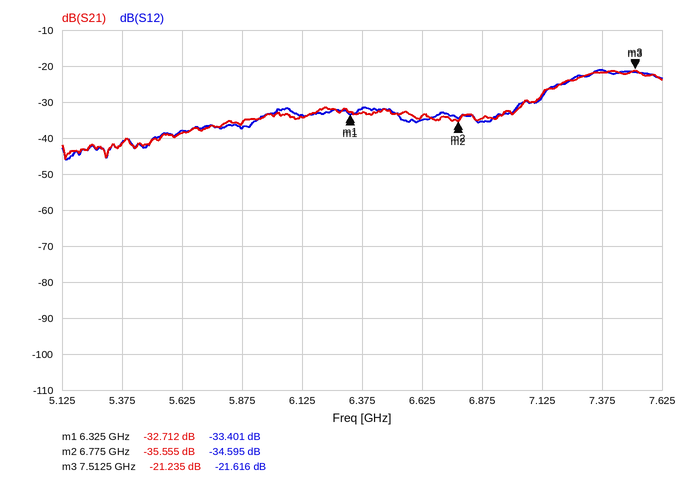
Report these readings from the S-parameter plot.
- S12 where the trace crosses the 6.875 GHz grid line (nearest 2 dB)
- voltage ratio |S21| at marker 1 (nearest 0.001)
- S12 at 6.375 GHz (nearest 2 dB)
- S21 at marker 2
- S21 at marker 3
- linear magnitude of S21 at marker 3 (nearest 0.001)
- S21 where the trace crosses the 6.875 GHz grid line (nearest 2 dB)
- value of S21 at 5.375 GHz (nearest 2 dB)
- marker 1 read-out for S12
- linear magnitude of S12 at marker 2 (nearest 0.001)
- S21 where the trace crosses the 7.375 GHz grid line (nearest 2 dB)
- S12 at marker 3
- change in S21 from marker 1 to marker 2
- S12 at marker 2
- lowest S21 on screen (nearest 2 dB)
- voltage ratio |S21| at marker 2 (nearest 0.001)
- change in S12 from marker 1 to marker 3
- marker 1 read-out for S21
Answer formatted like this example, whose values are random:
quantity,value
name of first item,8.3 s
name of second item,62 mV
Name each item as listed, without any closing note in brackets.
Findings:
quantity,value
S12 where the trace crosses the 6.875 GHz grid line,-36 dB
voltage ratio |S21| at marker 1,0.023
S12 at 6.375 GHz,-32 dB
S21 at marker 2,-35.555 dB
S21 at marker 3,-21.235 dB
linear magnitude of S21 at marker 3,0.087
S21 where the trace crosses the 6.875 GHz grid line,-34 dB
value of S21 at 5.375 GHz,-42 dB
marker 1 read-out for S12,-33.401 dB
linear magnitude of S12 at marker 2,0.019
S21 where the trace crosses the 7.375 GHz grid line,-22 dB
S12 at marker 3,-21.616 dB
change in S21 from marker 1 to marker 2,-2.843 dB
S12 at marker 2,-34.595 dB
lowest S21 on screen,-46 dB
voltage ratio |S21| at marker 2,0.017
change in S12 from marker 1 to marker 3,11.785 dB
marker 1 read-out for S21,-32.712 dB
